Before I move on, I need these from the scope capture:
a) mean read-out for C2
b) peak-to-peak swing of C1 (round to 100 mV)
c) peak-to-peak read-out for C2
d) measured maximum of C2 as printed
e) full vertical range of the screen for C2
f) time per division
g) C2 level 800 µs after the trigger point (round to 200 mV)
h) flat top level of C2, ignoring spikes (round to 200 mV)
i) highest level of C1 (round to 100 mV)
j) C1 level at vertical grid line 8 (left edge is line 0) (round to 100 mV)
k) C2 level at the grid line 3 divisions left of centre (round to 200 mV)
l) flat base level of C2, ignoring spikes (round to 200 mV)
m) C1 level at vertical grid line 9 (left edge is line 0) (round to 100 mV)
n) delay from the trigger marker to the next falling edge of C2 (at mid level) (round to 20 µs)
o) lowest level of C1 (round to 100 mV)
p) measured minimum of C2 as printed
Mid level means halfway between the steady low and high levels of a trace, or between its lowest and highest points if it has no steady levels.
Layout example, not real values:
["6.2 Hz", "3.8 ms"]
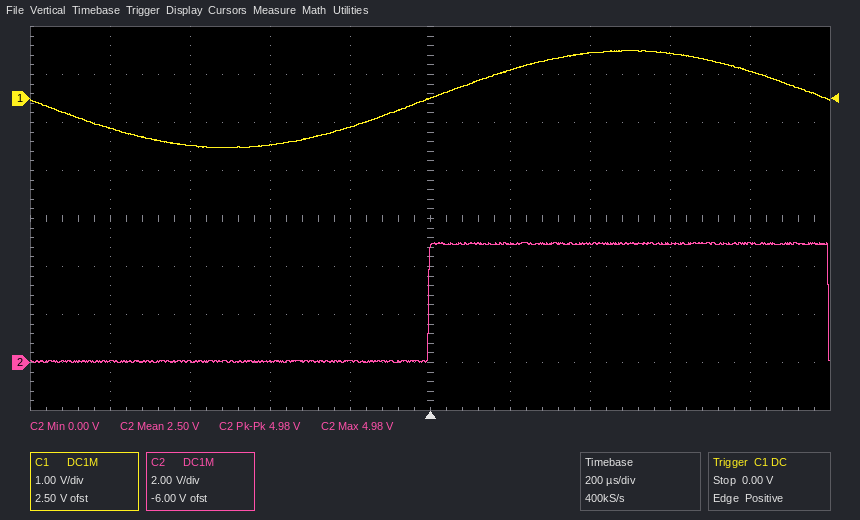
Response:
["2.50 V", "2.0 V", "4.98 V", "4.98 V", "16 V", "200 µs", "5.0 V", "5.0 V", "1.0 V", "900 mV", "0.0 V", "0.0 V", "600 mV", "1.00 ms", "-1.0 V", "0.00 V"]
